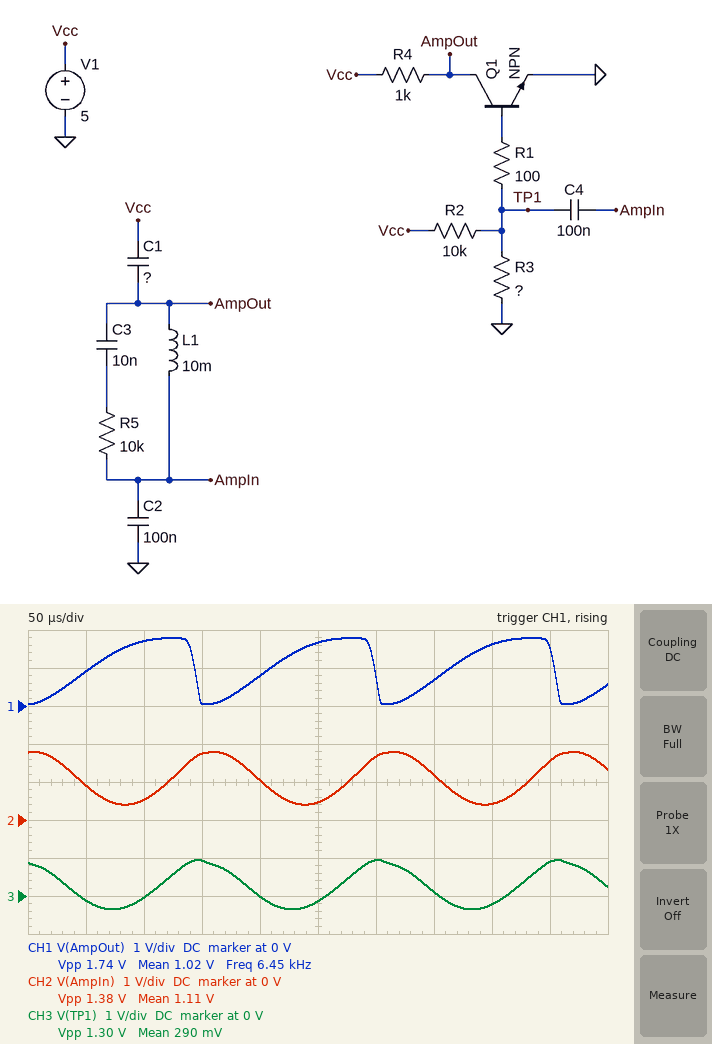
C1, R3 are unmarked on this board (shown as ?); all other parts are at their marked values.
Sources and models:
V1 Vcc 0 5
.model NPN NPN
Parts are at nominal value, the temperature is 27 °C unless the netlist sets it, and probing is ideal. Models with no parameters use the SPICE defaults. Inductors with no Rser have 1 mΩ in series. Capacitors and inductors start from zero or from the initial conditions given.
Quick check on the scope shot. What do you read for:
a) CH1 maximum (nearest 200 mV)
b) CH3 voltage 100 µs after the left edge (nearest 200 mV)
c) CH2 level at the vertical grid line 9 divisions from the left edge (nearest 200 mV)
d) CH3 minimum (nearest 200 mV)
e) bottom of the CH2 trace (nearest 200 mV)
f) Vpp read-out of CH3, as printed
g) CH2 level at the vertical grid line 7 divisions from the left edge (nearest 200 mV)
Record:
1.8 V
0 V
1.6 V
-400 mV
400 mV
1.30 V
1.2 V
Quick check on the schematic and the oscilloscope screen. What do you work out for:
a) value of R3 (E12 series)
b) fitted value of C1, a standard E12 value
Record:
680 Ω
330 nF
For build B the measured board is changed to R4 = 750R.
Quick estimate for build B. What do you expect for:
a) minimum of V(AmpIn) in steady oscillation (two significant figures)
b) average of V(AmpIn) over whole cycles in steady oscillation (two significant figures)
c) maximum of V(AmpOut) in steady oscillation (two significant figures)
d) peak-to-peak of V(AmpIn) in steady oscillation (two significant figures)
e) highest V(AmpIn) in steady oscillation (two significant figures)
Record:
550 mV
1.3 V
2.1 V
1.5 V
2.0 V
